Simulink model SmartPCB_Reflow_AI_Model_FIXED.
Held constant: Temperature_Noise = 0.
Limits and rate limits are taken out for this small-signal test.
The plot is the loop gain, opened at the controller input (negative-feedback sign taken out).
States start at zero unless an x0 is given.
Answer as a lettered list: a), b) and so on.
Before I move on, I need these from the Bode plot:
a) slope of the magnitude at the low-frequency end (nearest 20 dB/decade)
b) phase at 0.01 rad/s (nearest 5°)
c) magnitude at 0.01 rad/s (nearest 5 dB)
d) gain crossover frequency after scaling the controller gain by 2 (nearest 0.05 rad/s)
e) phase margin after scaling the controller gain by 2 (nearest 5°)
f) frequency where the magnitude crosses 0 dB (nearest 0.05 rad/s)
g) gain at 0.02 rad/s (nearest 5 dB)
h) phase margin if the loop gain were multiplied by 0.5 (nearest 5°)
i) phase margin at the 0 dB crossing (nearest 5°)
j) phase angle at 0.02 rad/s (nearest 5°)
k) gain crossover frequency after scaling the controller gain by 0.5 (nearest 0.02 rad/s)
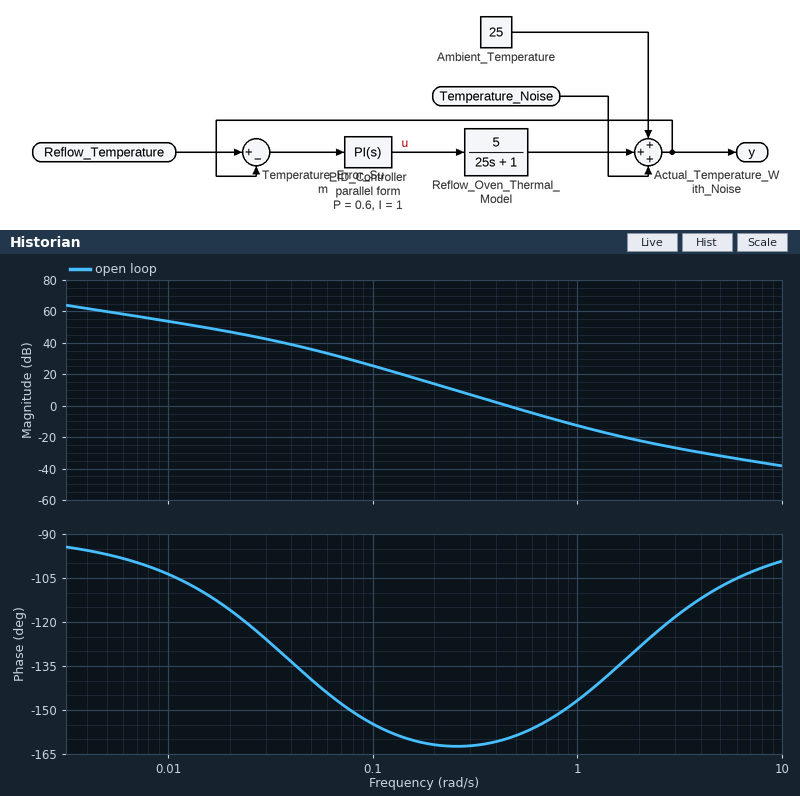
a) -20 dB/decade
b) -105°
c) 55 dB
d) 0.65 rad/s
e) 25°
f) 0.45 rad/s
g) 45 dB
h) 20°
i) 20°
j) -115°
k) 0.32 rad/s
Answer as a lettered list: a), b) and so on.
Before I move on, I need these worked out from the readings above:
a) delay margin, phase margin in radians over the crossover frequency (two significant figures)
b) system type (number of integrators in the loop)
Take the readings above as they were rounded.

a) 0.78 s
b) 1
